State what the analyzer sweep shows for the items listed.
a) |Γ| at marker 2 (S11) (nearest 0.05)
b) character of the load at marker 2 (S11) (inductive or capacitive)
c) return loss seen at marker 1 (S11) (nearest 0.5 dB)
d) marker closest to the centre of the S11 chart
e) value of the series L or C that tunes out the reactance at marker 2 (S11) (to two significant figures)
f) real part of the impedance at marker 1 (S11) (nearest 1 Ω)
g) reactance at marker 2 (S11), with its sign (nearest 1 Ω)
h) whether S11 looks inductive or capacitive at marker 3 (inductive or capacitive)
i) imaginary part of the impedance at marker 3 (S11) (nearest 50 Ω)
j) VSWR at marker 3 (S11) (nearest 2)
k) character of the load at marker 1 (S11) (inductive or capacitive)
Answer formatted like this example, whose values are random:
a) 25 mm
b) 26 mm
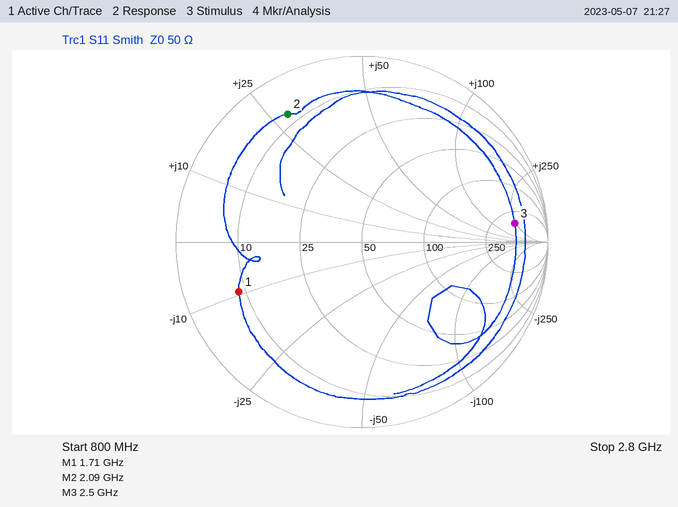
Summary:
a) 0.80
b) inductive
c) 3.0 dB
d) marker 1
e) 2.7 pF
f) 9 Ω
g) +28 Ω
h) inductive
i) +250 Ω
j) 10
k) capacitive
